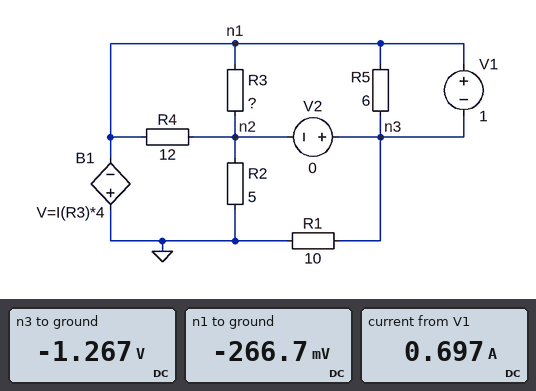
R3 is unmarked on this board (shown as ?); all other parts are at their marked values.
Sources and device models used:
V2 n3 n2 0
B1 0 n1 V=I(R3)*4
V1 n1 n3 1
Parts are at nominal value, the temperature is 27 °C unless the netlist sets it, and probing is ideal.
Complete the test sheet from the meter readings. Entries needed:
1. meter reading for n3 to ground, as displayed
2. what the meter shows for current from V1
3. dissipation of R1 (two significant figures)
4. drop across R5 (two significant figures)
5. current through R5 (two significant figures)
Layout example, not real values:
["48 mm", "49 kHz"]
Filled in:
["-1.267 V", "0.697 A", "160 mW", "1.0 V", "170 mA"]
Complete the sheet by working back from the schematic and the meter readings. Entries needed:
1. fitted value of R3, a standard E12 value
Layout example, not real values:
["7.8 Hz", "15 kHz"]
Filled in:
["15 Ω"]
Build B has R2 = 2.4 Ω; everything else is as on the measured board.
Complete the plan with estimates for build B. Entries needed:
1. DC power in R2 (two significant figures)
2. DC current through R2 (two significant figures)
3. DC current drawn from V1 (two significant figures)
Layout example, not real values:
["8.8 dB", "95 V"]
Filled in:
["670 mW", "530 mA", "970 mA"]
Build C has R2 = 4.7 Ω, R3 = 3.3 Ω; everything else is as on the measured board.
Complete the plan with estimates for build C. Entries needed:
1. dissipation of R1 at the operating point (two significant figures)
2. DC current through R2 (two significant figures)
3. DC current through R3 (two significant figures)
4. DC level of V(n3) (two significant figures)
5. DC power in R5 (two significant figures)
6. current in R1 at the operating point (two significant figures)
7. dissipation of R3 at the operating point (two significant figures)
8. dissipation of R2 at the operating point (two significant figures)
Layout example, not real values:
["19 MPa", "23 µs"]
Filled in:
["490 mW", "470 mA", "300 mA", "-2.2 V", "170 mW", "220 mA", "300 mW", "1.0 W"]
